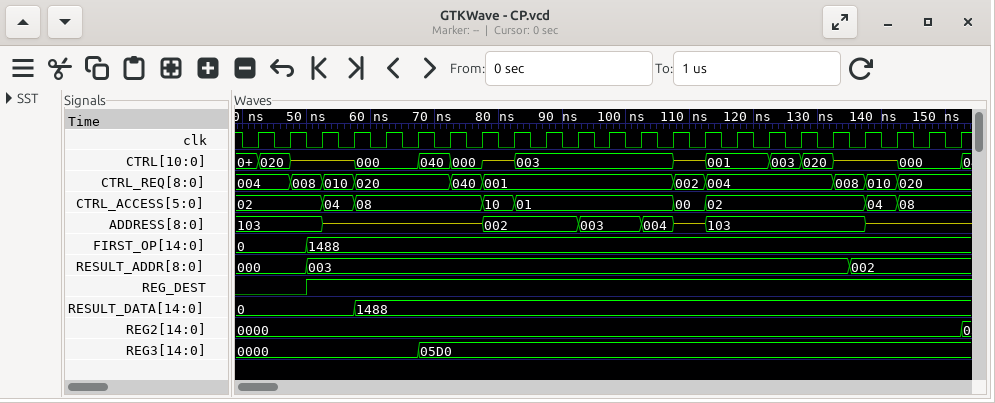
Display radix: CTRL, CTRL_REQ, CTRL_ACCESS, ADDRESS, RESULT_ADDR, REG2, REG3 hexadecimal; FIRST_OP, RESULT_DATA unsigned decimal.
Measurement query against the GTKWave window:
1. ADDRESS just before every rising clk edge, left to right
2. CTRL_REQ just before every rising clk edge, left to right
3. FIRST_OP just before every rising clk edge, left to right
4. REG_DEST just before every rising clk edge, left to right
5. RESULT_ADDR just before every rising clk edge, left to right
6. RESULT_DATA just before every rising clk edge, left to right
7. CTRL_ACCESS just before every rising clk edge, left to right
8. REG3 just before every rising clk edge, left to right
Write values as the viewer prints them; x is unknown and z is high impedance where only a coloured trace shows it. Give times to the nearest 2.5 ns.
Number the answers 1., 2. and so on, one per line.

1. 103, 103, 103, z, z, z, z, z, 002, 002, 002, 003, 003, 004, z, 103, 103, 103, 103, 103, z, z, z
2. 004, 004, 008, 010, 020, 020, 020, 040, 001, 001, 001, 001, 001, 001, 002, 004, 004, 004, 004, 008, 010, 020, 020
3. 0, 0, 1488, 1488, 1488, 1488, 1488, 1488, 1488, 1488, 1488, 1488, 1488, 1488, 1488, 1488, 1488, 1488, 1488, 1488, 1488, 1488, 1488
4. 0 0 1 1 1 1 1 1 1 1 1 1 1 1 1 1 1 1 1 1 1 1 1
5. 000, 000, 003, 003, 003, 003, 003, 003, 003, 003, 003, 003, 003, 003, 003, 003, 003, 003, 003, 002, 002, 002, 002
6. 0, 0, 0, 0, 1488, 1488, 1488, 1488, 1488, 1488, 1488, 1488, 1488, 1488, 1488, 1488, 1488, 1488, 1488, 1488, 1488, 1488, 1488
7. 02, 02, 02, 04, 08, 08, 08, 08, 10, 01, 01, 01, 01, 01, 00, 02, 02, 02, 02, 02, 04, 08, 08
8. 0000, 0000, 0000, 0000, 0000, 0000, 05D0, 05D0, 05D0, 05D0, 05D0, 05D0, 05D0, 05D0, 05D0, 05D0, 05D0, 05D0, 05D0, 05D0, 05D0, 05D0, 05D0
